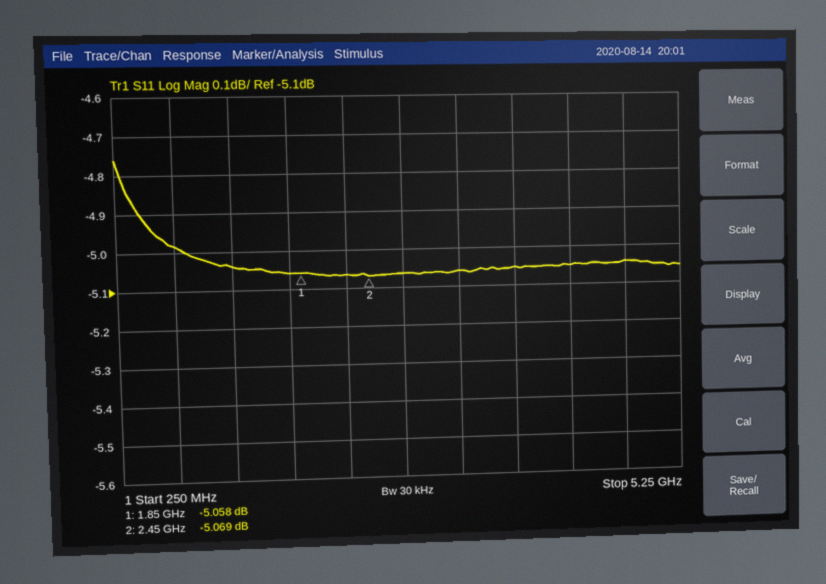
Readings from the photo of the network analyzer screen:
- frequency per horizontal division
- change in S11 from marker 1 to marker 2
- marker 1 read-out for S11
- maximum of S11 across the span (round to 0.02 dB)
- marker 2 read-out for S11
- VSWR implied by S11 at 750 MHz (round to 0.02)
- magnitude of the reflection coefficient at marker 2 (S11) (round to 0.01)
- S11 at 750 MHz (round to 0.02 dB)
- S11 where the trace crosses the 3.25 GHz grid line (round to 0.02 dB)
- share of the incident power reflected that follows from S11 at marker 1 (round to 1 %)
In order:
500 MHz
-0.011 dB
-5.058 dB
-4.76 dB
-5.069 dB
3.58
0.56
-4.98 dB
-5.06 dB
31 %
